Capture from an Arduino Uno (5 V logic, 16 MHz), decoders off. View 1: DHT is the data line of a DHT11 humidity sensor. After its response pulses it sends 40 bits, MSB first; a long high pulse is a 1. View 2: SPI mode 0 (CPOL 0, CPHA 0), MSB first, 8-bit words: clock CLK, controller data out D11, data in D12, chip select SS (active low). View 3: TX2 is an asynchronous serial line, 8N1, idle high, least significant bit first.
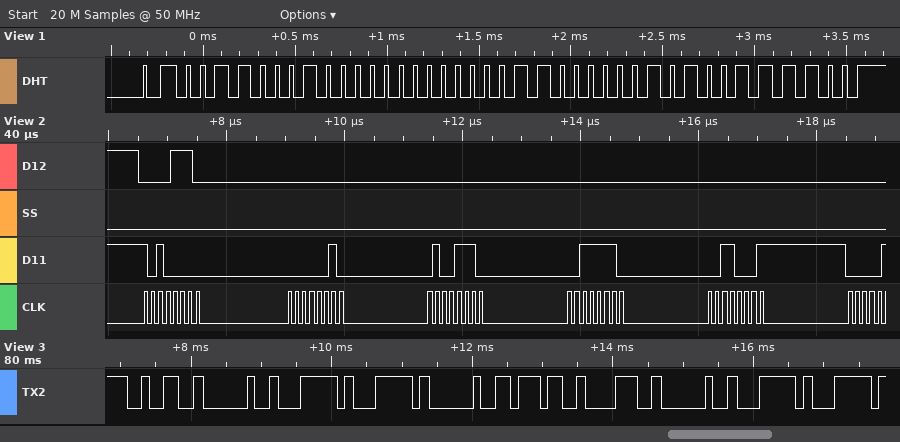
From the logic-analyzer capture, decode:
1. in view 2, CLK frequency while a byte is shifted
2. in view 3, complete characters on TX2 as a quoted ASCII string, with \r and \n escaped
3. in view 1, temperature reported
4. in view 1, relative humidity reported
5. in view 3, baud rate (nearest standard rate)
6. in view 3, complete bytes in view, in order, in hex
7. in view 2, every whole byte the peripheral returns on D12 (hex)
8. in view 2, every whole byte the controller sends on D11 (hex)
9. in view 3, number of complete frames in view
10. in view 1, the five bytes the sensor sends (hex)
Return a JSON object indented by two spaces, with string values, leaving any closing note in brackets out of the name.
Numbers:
{
  "in view 2, CLK frequency while a byte is shifted": "8 MHz",
  "in view 3, complete characters on TX2 as a quoted ASCII string, with \\r and \\n escaped": "\"2 || 78 ||\"",
  "in view 1, temperature reported": "6.5 °C",
  "in view 1, relative humidity reported": "49 %",
  "in view 3, baud rate": "9600 baud",
  "in view 3, complete bytes in view, in order, in hex": "32 20 7C 7C 20 37 38 20 7C 7C",
  "in view 2, every whole byte the peripheral returns on D12": "0x0E 0x00 0x00 0x00 0x00",
  "in view 2, every whole byte the controller sends on D11": "0xA0 0x02 0x4E 0x3E 0x31",
  "in view 3, number of complete frames in view": "10",
  "in view 1, the five bytes the sensor sends": "31 00 06 05 3C"
}
